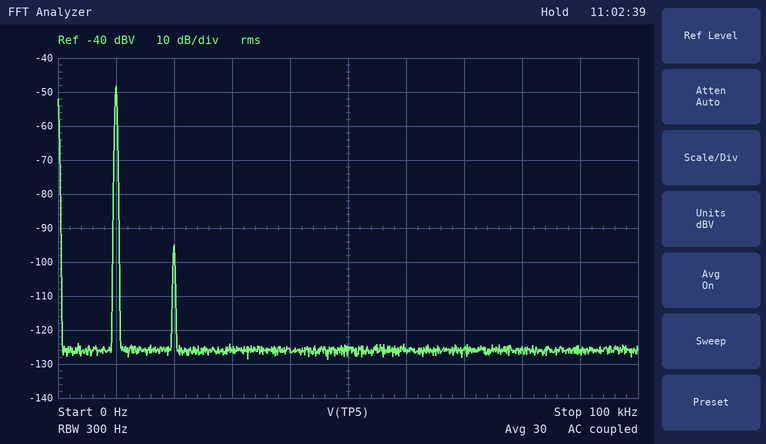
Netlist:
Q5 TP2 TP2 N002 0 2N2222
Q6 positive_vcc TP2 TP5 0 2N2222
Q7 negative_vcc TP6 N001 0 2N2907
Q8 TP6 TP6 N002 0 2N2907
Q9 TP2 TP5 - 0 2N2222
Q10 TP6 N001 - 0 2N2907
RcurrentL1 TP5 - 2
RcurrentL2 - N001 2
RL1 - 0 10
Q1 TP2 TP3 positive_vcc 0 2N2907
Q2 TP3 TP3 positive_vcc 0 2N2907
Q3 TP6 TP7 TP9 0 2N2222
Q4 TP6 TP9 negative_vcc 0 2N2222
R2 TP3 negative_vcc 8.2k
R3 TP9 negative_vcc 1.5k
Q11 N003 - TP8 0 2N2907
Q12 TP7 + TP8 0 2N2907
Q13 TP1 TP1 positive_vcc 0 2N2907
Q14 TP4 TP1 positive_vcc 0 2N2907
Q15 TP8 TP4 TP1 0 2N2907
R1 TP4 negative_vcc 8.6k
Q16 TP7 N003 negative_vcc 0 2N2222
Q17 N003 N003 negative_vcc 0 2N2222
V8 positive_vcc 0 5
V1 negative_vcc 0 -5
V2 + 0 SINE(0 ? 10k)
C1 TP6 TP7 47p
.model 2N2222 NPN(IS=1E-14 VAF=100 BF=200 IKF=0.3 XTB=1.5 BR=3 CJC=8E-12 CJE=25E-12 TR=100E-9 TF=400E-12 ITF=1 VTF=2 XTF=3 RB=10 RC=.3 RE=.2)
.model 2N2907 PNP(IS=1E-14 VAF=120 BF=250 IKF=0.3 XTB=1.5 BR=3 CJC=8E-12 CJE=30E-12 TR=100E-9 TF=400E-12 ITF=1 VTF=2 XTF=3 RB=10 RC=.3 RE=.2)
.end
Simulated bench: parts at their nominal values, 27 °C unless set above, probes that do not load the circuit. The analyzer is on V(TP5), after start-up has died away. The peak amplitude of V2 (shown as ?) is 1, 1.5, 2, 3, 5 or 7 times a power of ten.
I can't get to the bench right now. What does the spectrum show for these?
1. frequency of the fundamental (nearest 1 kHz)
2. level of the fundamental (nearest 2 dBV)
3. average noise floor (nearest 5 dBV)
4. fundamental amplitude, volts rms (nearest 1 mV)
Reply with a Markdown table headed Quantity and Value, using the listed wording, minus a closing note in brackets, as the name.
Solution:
| Quantity | Value |
|---|---|
| frequency of the fundamental | 10 kHz |
| level of the fundamental | -48 dBV |
| average noise floor | -125 dBV |
| fundamental amplitude, volts rms | 4 mV |
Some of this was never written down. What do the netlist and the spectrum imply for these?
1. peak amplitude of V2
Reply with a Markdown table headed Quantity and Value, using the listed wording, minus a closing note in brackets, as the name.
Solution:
| Quantity | Value |
|---|---|
| peak amplitude of V2 | 5 mV |
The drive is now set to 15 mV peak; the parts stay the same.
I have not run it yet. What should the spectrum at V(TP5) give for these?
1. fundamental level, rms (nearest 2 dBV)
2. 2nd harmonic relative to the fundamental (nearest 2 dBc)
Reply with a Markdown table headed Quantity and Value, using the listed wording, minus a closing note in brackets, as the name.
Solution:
| Quantity | Value |
|---|---|
| fundamental level, rms | -38 dBV |
| 2nd harmonic relative to the fundamental | -38 dBc |
